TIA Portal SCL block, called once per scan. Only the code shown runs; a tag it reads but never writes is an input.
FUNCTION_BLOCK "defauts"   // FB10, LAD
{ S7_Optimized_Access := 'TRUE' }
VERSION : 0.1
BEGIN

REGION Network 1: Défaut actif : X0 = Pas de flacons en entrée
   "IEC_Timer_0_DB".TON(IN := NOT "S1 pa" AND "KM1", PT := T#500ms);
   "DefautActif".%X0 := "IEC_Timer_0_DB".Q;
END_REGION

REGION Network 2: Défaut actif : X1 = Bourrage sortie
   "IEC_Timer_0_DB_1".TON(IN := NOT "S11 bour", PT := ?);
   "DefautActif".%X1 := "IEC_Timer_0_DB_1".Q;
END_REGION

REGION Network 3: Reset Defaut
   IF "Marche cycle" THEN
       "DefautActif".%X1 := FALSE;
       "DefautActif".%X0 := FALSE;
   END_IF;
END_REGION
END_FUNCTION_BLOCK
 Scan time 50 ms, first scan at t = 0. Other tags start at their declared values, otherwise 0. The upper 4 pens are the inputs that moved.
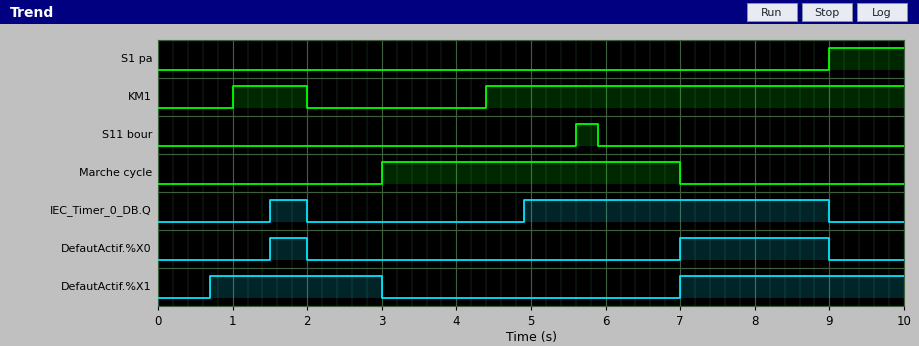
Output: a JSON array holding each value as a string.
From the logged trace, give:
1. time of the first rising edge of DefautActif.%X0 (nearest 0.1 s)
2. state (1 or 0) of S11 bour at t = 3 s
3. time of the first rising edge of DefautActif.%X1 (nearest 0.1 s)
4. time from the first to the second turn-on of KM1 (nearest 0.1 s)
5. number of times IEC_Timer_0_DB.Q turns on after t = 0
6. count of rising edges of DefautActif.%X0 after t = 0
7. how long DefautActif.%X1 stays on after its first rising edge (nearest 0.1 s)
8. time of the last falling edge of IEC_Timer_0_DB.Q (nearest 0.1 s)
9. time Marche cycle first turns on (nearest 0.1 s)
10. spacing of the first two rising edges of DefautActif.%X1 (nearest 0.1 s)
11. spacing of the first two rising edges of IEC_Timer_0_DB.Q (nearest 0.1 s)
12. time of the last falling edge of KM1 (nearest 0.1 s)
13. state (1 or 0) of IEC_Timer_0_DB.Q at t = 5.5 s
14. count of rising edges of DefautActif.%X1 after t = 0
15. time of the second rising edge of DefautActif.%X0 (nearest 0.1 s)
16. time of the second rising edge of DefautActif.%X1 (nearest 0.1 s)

["1.5 s", "0", "0.7 s", "3.4 s", "2", "2", "2.3 s", "9.0 s", "3.0 s", "6.3 s", "3.4 s", "2.0 s", "1", "2", "7.0 s", "7.0 s"]
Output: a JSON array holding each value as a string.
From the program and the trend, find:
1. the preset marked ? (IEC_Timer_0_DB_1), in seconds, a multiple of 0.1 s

["0.7 s"]
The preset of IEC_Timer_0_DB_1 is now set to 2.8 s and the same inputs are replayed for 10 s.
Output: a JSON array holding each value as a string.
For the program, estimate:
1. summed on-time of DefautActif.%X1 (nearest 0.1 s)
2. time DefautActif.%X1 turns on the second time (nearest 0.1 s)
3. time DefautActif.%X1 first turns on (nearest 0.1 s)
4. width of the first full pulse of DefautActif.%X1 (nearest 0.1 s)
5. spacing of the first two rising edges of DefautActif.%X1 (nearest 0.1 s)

["1.5 s", "8.7 s", "2.8 s", "0.2 s", "5.9 s"]
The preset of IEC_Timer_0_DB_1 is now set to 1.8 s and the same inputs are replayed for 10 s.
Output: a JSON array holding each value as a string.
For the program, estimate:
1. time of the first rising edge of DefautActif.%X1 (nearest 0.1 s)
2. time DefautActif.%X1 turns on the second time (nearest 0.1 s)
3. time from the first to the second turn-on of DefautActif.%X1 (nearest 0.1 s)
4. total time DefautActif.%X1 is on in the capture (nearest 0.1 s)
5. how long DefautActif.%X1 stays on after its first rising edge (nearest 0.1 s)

["1.8 s", "7.7 s", "5.9 s", "3.5 s", "1.2 s"]
